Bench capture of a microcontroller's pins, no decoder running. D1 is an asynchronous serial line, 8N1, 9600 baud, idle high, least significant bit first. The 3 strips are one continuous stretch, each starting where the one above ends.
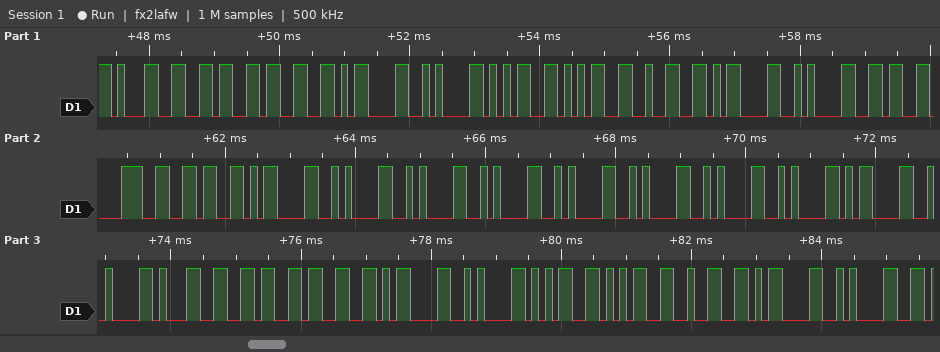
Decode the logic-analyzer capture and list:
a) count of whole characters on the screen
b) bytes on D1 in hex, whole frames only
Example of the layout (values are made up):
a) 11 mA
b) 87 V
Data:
a) 33
b) 0x31 0x36 0x33 0x0D 0x0A 0x35 0x35 0x32 0x0D 0x0A 0x36 0x38 0x36 0x0D 0x0A 0x0A 0x0A 0x0A 0x0A 0x0A 0x0A 0x0D 0x0A 0x31 0x36 0x33 0x0D 0x0A 0x35 0x35 0x32 0x0D 0x0A
